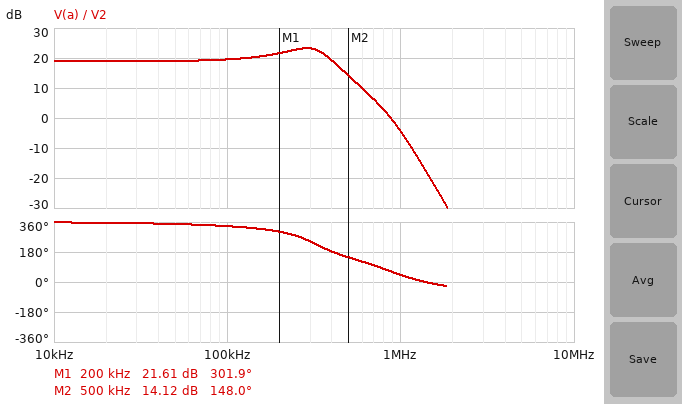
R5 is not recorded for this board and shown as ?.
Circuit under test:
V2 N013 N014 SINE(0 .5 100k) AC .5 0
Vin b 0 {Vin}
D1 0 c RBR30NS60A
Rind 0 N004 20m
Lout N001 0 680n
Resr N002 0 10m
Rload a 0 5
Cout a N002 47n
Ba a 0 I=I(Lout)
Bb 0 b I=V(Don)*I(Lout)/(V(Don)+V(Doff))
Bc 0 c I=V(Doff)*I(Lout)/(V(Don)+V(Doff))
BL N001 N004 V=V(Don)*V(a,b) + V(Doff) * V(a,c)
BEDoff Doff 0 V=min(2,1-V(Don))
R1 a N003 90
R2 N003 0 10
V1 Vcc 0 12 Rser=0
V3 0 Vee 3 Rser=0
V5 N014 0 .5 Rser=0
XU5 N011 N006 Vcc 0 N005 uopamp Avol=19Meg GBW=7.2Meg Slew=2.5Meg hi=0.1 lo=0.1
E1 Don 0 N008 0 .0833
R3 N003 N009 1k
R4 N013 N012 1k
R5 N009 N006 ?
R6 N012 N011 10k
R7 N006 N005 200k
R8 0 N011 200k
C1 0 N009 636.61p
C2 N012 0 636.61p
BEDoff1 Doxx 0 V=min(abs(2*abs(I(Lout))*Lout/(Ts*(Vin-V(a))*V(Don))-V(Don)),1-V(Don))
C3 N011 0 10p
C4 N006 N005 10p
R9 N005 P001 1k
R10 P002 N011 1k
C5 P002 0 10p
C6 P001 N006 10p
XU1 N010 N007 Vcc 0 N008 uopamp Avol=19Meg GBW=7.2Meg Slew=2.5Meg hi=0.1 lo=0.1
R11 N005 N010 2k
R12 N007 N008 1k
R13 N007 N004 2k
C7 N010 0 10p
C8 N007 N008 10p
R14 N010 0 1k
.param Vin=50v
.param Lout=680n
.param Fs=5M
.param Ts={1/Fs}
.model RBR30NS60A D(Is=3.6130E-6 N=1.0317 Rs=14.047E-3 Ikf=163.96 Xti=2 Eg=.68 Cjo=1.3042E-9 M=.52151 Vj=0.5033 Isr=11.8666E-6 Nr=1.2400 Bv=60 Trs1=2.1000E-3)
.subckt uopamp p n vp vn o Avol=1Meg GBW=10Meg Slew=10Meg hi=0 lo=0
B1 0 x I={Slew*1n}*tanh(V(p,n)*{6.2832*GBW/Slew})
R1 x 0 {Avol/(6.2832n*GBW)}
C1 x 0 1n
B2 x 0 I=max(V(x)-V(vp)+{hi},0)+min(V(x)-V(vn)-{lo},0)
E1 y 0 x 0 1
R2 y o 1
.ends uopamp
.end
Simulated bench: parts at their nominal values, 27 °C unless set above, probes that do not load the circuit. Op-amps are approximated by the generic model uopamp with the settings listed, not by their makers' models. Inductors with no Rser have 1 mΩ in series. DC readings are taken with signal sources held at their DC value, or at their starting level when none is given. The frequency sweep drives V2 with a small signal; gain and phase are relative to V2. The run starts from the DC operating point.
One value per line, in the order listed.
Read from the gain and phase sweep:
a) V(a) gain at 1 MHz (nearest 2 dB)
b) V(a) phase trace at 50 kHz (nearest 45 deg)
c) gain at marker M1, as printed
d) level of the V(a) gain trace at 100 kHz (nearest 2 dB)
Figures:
-4 dB
360 deg
21.61 dB
20 dB
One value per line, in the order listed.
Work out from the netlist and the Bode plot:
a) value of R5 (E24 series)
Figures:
3.3 kΩ
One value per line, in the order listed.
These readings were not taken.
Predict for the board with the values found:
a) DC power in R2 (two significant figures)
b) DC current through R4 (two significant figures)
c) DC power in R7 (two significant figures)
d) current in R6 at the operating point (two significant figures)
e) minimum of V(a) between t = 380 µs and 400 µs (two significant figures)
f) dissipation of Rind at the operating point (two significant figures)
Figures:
19 mW
2.4 µA
16 µW
2.4 µA
120 mV
17 mW
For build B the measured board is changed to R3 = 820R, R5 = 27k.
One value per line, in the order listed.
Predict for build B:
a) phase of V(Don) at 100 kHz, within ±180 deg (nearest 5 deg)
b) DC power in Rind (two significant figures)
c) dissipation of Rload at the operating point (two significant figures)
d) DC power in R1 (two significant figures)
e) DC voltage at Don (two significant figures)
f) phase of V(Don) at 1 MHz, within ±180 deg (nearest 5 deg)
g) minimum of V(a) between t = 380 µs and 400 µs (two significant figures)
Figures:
-55 deg
8.5 mW
1.9 W
86 mW
68 mV
-165 deg
580 mV
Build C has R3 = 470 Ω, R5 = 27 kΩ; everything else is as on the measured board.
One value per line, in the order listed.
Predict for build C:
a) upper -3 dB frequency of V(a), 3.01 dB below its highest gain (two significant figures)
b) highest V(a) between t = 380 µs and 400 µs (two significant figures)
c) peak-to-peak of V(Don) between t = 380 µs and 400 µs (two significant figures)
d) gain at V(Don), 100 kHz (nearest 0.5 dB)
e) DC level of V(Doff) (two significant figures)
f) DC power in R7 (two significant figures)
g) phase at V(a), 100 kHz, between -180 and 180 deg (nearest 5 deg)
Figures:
110 kHz
5.5 V
96 mV
-20.5 dB
930 mV
7.0 µW
-60 deg
